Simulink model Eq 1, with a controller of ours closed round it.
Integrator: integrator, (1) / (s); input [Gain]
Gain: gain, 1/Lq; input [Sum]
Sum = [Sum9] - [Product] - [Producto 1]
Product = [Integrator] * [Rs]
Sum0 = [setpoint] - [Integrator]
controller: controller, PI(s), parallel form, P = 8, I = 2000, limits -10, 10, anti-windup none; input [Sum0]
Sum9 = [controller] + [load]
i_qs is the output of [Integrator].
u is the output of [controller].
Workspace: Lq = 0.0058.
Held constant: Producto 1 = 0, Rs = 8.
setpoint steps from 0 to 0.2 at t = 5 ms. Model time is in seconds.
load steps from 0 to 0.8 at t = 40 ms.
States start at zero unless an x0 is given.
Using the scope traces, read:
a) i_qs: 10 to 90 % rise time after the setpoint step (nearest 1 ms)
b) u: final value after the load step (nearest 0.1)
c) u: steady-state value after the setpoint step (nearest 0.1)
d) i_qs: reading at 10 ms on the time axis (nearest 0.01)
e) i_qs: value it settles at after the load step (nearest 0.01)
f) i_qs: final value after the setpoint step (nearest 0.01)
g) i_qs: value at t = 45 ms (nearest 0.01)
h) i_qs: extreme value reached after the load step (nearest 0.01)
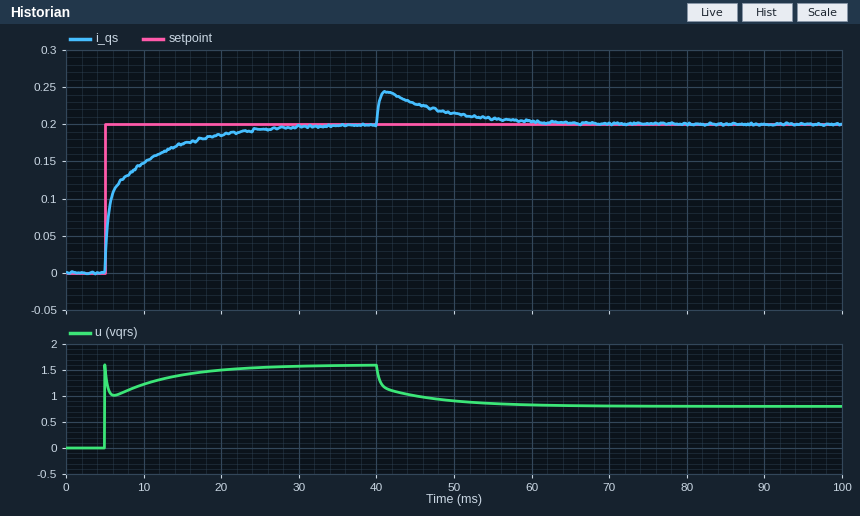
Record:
12 ms
0.8
1.6
0.15
0.20
0.20
0.23
0.24
